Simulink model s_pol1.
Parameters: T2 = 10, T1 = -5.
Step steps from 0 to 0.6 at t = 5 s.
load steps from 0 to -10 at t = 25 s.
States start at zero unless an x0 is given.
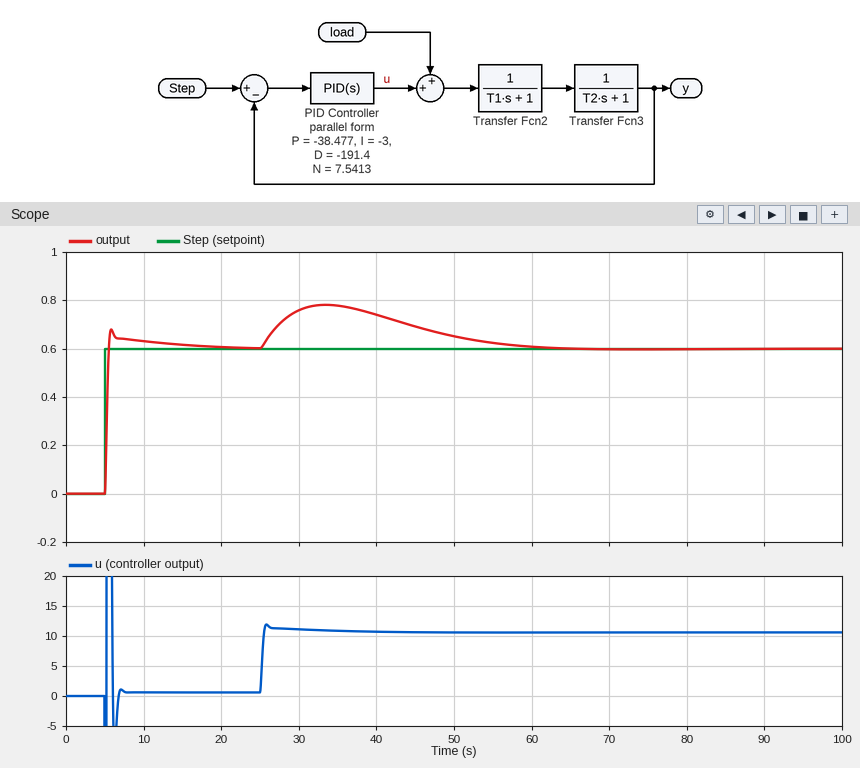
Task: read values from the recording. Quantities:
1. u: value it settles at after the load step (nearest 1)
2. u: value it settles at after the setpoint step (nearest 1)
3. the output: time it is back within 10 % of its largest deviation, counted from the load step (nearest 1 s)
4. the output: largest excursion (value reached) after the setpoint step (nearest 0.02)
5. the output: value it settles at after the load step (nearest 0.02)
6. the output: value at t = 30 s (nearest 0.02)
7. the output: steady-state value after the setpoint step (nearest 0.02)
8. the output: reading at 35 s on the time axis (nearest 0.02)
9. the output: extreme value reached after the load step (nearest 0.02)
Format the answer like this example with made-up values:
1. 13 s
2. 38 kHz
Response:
1. 11
2. 1
3. 32 s
4. 0.68
5. 0.60
6. 0.76
7. 0.60
8. 0.78
9. 0.78
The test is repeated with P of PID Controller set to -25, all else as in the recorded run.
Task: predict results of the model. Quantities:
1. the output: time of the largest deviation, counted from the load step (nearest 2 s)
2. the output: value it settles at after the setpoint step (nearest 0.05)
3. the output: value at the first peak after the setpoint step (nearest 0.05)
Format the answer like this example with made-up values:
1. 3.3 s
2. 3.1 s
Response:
1. 10 s
2. 0.60
3. 0.65
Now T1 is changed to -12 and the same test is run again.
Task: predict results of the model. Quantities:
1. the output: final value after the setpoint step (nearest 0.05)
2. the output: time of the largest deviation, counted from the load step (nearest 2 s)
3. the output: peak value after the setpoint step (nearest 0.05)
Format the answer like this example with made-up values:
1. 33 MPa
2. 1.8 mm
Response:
1. 0.60
2. 8 s
3. 0.65
